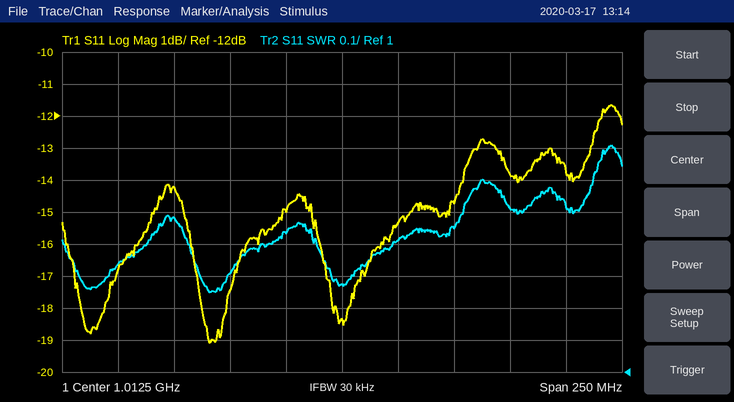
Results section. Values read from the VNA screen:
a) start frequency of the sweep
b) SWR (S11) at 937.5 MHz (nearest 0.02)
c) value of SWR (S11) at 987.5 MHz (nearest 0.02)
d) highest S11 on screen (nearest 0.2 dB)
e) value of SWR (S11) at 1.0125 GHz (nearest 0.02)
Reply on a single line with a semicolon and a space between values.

887.5 MHz; 1.48; 1.44; -11.6 dB; 1.28
